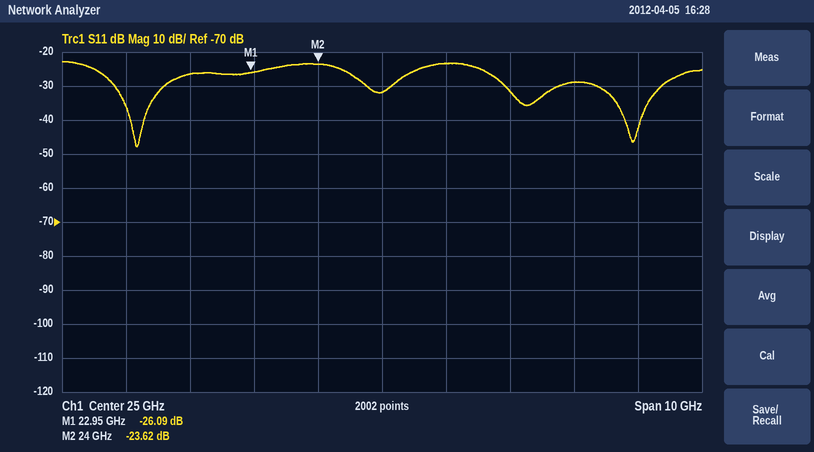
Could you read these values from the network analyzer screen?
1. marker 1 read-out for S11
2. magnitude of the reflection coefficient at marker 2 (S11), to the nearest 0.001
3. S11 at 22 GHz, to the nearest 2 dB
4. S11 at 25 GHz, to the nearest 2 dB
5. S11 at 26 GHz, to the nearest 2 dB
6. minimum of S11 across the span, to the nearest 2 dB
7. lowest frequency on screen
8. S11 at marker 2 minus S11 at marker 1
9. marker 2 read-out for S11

-26.09 dB
0.066
-26 dB
-32 dB
-24 dB
-48 dB
20 GHz
2.47 dB
-23.62 dB
